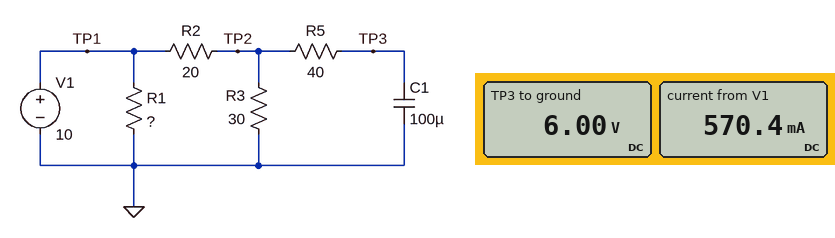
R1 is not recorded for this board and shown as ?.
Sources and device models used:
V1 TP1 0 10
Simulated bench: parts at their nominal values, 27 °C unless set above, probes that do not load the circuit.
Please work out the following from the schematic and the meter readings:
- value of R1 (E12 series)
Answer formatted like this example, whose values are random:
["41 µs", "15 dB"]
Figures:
["27 Ω"]
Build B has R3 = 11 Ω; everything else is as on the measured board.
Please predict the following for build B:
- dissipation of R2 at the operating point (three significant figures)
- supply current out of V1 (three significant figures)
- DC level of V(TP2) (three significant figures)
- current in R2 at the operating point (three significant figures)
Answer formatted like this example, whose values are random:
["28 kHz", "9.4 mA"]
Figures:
["2.08 W", "693 mA", "3.55 V", "323 mA"]
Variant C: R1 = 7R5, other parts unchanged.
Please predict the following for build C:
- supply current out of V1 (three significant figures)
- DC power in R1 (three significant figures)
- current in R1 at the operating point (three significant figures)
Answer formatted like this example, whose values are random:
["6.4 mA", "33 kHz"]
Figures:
["1.53 A", "13.3 W", "1.33 A"]
